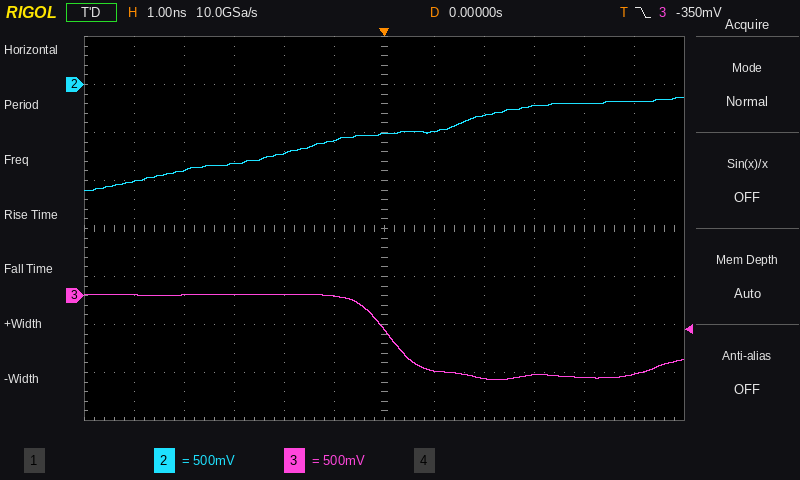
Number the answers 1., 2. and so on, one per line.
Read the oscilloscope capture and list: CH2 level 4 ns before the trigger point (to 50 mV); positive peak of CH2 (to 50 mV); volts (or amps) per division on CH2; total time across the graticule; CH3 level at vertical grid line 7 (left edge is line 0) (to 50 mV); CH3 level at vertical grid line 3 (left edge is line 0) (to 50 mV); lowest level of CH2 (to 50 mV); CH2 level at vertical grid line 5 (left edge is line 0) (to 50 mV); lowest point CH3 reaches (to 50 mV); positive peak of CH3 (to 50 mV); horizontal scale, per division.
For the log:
1. -900 mV
2. -150 mV
3. 500 mV
4. 12 ns
5. -800 mV
6. 0 mV
7. -1.10 V
8. -600 mV
9. -850 mV
10. 0 mV
11. 1 ns
